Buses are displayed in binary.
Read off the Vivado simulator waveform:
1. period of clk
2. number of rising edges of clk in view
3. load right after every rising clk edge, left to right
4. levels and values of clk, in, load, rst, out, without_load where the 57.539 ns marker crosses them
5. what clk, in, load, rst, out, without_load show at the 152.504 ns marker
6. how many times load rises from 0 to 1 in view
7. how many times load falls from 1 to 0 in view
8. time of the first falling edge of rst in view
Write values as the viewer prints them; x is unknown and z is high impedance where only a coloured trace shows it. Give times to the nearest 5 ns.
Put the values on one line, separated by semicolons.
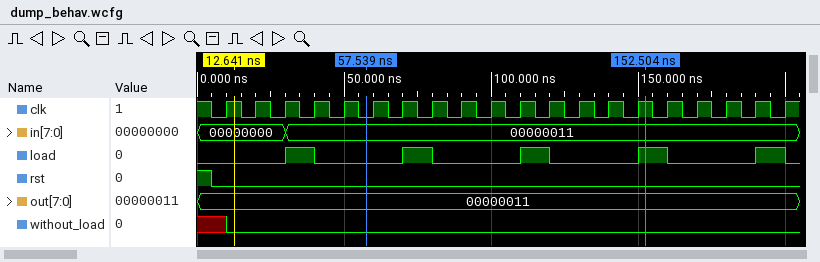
10 ns; 20; 0 0 1 0 0 0 1 0 0 0 1 0 0 0 1 0 0 0 1 0; clk=0, in=00000011, load=0, rst=0, out=00000011, without_load=0; clk=1, in=00000011, load=1, rst=0, out=00000011, without_load=0; 5; 5; 5 ns
